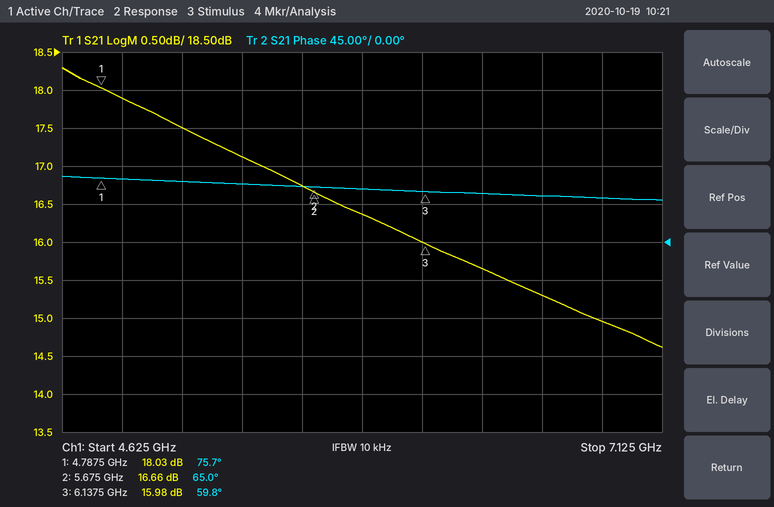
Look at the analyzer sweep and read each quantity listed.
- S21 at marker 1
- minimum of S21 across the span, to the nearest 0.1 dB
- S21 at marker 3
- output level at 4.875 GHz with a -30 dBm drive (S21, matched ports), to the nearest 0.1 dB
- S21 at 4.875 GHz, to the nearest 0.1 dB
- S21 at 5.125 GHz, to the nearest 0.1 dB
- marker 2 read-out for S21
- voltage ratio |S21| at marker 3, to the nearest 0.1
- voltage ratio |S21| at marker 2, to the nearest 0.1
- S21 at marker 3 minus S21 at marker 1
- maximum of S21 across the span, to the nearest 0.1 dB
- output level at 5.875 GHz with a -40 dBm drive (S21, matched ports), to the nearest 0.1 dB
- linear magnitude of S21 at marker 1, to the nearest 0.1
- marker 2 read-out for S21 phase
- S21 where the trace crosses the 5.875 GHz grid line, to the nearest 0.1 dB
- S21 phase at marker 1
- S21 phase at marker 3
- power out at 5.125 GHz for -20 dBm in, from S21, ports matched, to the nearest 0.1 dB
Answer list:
18.03 dB
14.6 dB
15.98 dB
-12.1 dBm
17.9 dB
17.5 dB
16.66 dB
6.3
6.8
-2.05 dB
18.3 dB
-23.6 dBm
8.0
65.0°
16.4 dB
75.7°
59.8°
-2.5 dBm
